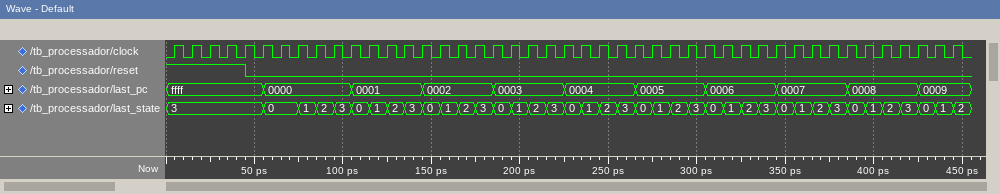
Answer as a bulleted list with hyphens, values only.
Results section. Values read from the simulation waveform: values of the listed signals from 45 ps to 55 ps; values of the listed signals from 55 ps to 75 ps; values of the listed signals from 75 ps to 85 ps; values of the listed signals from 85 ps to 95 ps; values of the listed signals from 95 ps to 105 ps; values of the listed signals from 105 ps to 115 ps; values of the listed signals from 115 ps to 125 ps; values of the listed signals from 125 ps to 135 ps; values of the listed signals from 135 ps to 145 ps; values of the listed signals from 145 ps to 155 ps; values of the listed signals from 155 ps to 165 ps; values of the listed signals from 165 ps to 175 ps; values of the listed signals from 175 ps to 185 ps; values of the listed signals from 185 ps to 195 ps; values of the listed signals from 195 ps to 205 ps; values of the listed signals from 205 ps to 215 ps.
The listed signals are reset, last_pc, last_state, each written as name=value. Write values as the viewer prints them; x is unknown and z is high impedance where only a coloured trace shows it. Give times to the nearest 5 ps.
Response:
- reset=0, last_pc=ffff, last_state=3
- reset=0, last_pc=0000, last_state=0
- reset=0, last_pc=0000, last_state=1
- reset=0, last_pc=0000, last_state=2
- reset=0, last_pc=0000, last_state=3
- reset=0, last_pc=0001, last_state=0
- reset=0, last_pc=0001, last_state=1
- reset=0, last_pc=0001, last_state=2
- reset=0, last_pc=0001, last_state=3
- reset=0, last_pc=0002, last_state=0
- reset=0, last_pc=0002, last_state=1
- reset=0, last_pc=0002, last_state=2
- reset=0, last_pc=0002, last_state=3
- reset=0, last_pc=0003, last_state=0
- reset=0, last_pc=0003, last_state=1
- reset=0, last_pc=0003, last_state=2
